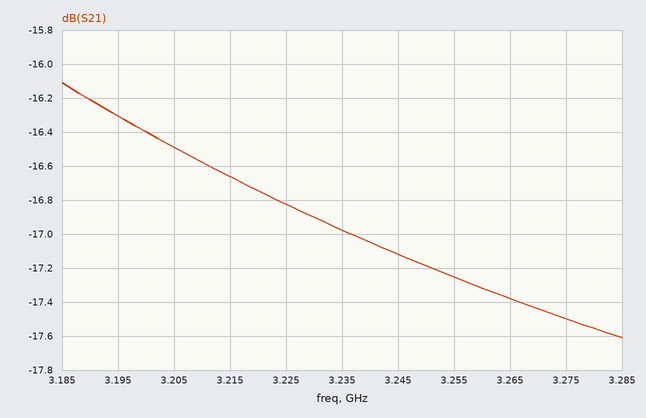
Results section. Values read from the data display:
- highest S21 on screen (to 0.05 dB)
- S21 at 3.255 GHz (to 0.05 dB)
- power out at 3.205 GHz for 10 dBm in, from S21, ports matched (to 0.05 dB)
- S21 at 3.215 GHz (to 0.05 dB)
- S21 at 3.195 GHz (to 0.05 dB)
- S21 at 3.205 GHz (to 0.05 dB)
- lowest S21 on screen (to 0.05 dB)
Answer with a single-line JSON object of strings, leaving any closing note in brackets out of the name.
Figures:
{"highest S21 on screen": "-16.10 dB", "S21 at 3.255 GHz": "-17.25 dB", "power out at 3.205 GHz for 10 dBm in, from S21, ports matched": "-6.50 dBm", "S21 at 3.215 GHz": "-16.65 dB", "S21 at 3.195 GHz": "-16.30 dB", "S21 at 3.205 GHz": "-16.50 dB", "lowest S21 on screen": "-17.60 dB"}
